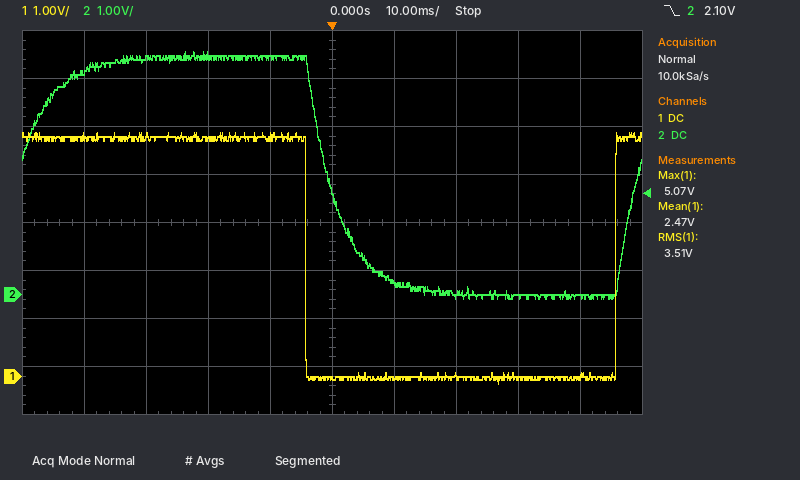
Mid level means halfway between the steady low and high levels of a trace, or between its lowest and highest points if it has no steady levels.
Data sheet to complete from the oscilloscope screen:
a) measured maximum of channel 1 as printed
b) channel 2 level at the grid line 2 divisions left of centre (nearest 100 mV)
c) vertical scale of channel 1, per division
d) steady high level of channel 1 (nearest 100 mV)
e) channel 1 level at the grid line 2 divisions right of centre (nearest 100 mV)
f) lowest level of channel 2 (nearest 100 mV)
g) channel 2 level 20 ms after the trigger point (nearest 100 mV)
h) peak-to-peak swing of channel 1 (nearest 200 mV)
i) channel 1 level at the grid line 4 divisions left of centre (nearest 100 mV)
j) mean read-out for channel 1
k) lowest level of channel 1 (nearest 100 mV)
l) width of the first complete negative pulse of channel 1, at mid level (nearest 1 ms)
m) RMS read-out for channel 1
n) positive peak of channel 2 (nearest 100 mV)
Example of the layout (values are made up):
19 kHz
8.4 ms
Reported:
5.07 V
5.0 V
1 V
5.0 V
0.0 V
-100 mV
0.0 V
5.2 V
5.0 V
2.47 V
-200 mV
50 ms
3.51 V
5.1 V
